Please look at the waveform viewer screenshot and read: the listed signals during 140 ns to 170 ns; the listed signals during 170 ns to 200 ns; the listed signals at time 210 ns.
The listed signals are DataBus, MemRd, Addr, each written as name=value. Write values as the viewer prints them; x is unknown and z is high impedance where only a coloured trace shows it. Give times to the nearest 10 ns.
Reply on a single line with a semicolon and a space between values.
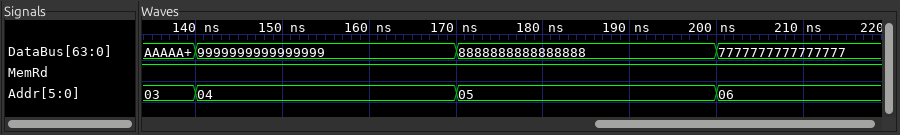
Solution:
DataBus=9999999999999999, MemRd=1, Addr=04; DataBus=8888888888888888, MemRd=1, Addr=05; DataBus=7777777777777777, MemRd=1, Addr=06
